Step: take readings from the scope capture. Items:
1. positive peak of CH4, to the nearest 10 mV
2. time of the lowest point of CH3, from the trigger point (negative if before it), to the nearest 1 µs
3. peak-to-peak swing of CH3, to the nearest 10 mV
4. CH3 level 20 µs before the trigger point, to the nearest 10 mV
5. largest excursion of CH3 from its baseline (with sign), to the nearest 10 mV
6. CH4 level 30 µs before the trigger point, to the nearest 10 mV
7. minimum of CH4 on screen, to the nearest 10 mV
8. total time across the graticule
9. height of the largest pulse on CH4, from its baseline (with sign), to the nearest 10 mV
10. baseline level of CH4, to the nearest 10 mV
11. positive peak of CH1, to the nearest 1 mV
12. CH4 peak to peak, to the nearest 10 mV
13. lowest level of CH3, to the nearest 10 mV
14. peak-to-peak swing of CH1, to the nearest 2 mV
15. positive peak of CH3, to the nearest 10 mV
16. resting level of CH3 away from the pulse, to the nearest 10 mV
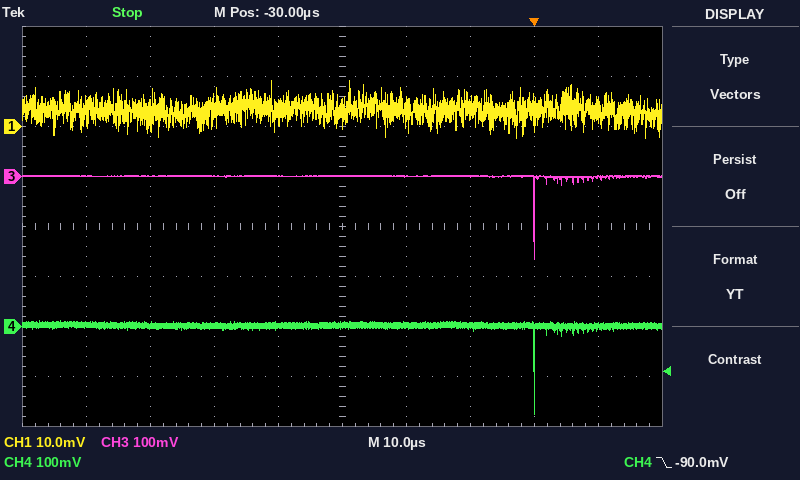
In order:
10 mV
0 µs
170 mV
0 mV
-170 mV
0 mV
-180 mV
100 µs
-180 mV
0 mV
9 mV
190 mV
-170 mV
12 mV
0 mV
0 mV
